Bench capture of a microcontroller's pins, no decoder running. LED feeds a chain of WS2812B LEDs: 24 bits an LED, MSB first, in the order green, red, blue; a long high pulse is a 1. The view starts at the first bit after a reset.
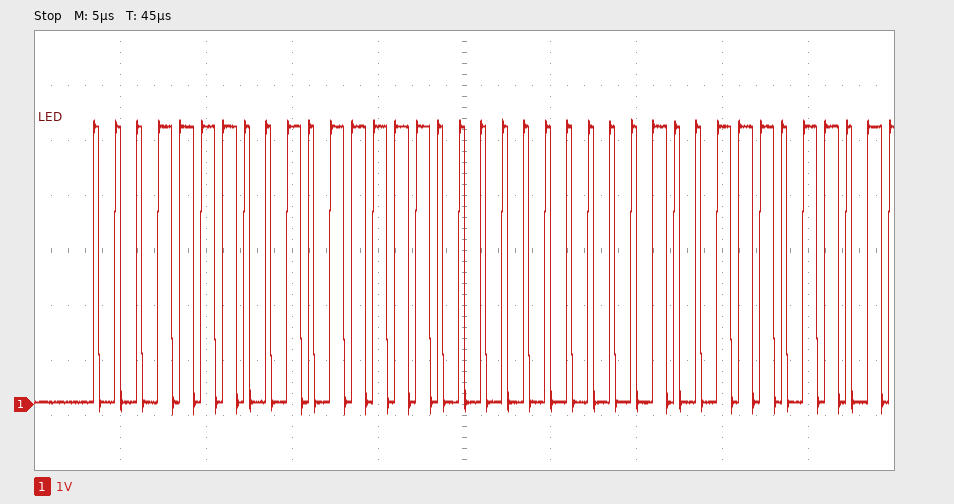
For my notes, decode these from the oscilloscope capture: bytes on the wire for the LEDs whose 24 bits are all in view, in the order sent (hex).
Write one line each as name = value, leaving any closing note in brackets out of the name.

bytes on the wire for the LEDs whose 24 bits are all in view, in the order sent = 1E 5F 00
